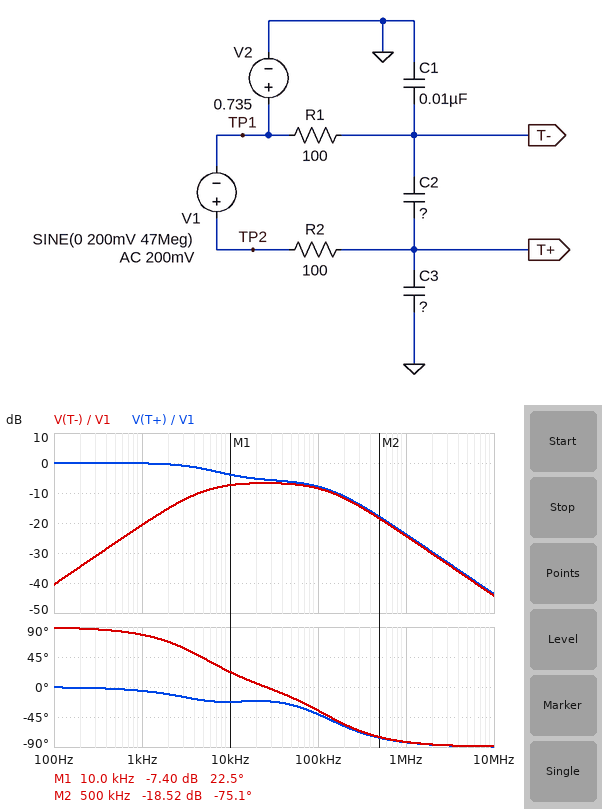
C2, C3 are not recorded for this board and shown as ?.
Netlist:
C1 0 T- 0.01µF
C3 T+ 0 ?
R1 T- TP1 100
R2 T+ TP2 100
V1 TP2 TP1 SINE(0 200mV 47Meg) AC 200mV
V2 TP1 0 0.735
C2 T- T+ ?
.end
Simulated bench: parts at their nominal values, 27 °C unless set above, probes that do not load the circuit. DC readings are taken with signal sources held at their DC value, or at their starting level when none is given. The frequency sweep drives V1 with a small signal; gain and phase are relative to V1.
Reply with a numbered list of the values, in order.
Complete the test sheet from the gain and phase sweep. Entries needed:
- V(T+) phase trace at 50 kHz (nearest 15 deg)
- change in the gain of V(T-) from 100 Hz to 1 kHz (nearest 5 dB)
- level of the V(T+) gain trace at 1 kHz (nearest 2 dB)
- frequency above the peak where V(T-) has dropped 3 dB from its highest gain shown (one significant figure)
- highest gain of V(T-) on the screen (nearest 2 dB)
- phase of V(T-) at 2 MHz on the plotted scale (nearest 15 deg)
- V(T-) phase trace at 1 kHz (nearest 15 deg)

1. -30 deg
2. 20 dB
3. 0 dB
4. 100 kHz
5. -6 dB
6. -90 deg
7. 75 deg
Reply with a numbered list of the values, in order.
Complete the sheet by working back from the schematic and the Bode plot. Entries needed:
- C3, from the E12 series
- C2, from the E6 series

1. 15 nF
2. 150 nF
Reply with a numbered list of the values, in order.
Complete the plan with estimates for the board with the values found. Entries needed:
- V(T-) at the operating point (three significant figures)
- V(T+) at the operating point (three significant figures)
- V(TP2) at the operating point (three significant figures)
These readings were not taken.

1. 735 mV
2. 735 mV
3. 735 mV
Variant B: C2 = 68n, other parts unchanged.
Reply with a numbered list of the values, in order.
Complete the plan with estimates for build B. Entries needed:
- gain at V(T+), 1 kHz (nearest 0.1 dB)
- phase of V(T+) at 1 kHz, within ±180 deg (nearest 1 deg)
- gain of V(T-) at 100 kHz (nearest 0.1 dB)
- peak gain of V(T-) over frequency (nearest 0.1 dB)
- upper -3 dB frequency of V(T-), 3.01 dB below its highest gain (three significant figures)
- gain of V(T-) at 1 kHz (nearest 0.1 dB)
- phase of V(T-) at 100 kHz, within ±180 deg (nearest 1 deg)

1. 0 dB
2. -3 deg
3. -8.9 dB
4. -7.5 dB
5. 148 kHz
6. -27.4 dB
7. -32 deg
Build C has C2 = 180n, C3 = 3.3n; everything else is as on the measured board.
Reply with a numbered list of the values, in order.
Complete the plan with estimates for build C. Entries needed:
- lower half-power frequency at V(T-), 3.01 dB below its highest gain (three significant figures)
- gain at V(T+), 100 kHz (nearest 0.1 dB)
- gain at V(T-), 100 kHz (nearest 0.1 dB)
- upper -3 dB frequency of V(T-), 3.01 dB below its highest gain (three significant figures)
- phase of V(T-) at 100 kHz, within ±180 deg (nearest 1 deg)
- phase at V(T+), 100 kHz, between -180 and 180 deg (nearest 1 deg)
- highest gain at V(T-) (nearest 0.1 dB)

1. 4.19 kHz
2. -6.4 dB
3. -6.9 dB
4. 249 kHz
5. -20 deg
6. -25 deg
7. -6.3 dB
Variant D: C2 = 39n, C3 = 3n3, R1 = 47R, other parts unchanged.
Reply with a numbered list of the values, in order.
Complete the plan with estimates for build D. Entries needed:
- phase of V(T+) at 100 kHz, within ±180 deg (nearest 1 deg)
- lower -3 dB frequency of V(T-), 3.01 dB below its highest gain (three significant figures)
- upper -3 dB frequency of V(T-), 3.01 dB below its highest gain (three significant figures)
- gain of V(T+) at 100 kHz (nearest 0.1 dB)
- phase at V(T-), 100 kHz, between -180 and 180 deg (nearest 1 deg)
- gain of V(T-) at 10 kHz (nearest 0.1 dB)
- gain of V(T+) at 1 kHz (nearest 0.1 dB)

1. -35 deg
2. 23.0 kHz
3. 424 kHz
4. -7.4 dB
5. 0 deg
6. -19.4 dB
7. 0 dB
